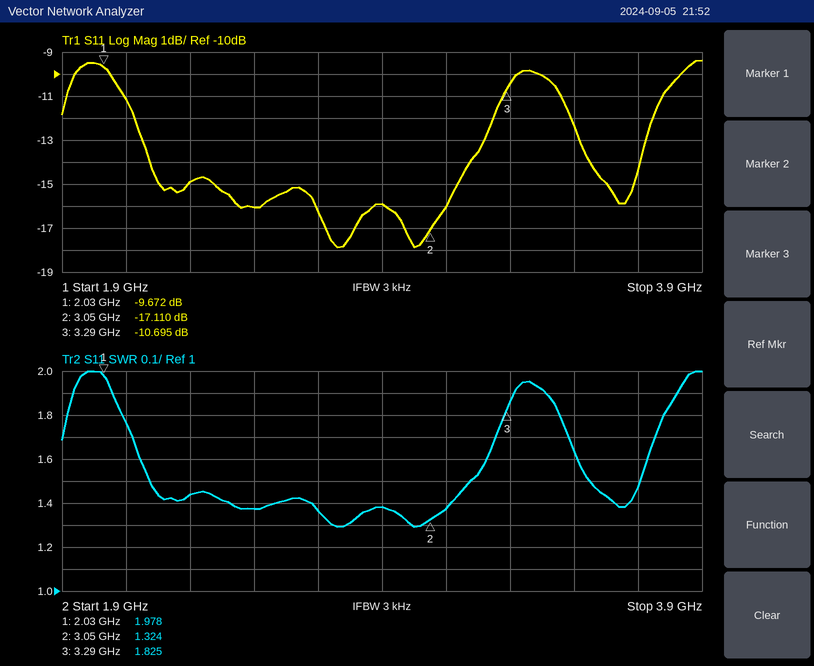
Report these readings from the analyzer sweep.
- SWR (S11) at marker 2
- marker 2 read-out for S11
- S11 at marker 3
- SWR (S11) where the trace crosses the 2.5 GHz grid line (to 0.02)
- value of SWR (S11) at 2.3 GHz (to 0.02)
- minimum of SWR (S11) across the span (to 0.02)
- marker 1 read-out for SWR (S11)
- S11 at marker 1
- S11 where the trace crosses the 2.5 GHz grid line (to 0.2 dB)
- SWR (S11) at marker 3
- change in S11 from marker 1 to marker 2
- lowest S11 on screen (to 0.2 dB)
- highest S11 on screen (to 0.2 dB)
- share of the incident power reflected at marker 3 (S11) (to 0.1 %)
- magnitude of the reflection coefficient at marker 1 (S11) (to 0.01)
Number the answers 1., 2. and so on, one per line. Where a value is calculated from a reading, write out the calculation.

1. 1.324
2. -17.110 dB
3. -10.695 dB
4. 1.38
5. 1.44
6. 1.30
7. 1.978
8. -9.672 dB
9. -16.0 dB
10. 1.825
11. -17.11 − (-9.672) = -7.438 dB
12. -17.8 dB
13. -9.4 dB
14. 10^(-10.695/10) ≈ 8.5 %
15. 10^(-9.672/20) ≈ 0.33
